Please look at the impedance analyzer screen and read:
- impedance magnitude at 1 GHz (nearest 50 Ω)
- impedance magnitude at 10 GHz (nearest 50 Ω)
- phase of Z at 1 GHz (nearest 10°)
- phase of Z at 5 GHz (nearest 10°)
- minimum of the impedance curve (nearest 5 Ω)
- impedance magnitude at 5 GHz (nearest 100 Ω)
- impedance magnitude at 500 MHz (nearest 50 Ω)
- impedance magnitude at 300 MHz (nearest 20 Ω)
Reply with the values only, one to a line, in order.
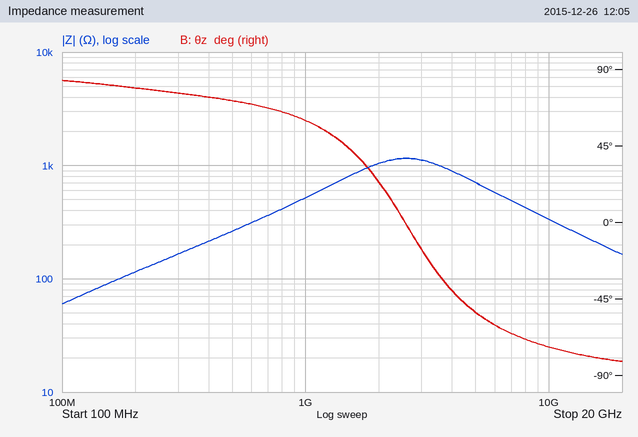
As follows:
500 Ω
350 Ω
60°
-50°
60 Ω
700 Ω
250 Ω
160 Ω
